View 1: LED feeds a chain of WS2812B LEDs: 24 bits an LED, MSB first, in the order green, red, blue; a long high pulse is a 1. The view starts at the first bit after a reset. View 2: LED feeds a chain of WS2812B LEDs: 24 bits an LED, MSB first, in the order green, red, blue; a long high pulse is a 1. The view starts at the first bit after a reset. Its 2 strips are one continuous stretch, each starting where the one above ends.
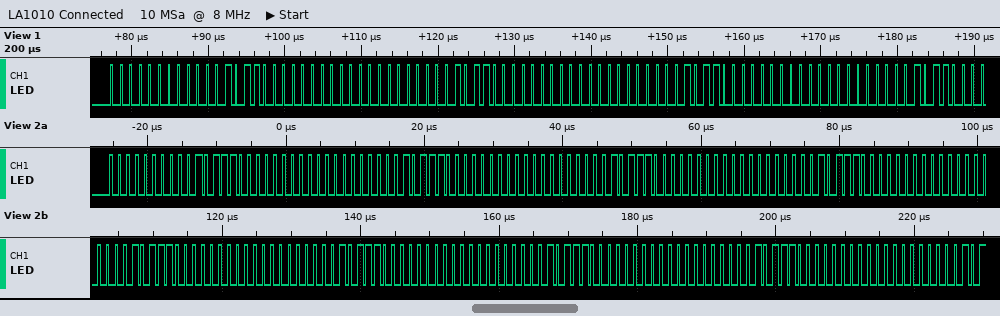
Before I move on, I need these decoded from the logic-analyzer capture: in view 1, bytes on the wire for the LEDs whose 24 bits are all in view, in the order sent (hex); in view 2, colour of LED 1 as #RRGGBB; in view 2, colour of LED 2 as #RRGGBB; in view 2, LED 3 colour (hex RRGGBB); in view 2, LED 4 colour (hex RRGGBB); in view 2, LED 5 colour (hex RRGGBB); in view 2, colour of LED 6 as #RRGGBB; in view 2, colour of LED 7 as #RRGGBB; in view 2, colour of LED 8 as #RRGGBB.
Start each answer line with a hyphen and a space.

- 00 0B 00 00 0B 00 00 0B 00
- #2E0000
- #2E0000
- #2E0000
- #2E0000
- #2E0000
- #2E0000
- #2E0000
- #2E0000
